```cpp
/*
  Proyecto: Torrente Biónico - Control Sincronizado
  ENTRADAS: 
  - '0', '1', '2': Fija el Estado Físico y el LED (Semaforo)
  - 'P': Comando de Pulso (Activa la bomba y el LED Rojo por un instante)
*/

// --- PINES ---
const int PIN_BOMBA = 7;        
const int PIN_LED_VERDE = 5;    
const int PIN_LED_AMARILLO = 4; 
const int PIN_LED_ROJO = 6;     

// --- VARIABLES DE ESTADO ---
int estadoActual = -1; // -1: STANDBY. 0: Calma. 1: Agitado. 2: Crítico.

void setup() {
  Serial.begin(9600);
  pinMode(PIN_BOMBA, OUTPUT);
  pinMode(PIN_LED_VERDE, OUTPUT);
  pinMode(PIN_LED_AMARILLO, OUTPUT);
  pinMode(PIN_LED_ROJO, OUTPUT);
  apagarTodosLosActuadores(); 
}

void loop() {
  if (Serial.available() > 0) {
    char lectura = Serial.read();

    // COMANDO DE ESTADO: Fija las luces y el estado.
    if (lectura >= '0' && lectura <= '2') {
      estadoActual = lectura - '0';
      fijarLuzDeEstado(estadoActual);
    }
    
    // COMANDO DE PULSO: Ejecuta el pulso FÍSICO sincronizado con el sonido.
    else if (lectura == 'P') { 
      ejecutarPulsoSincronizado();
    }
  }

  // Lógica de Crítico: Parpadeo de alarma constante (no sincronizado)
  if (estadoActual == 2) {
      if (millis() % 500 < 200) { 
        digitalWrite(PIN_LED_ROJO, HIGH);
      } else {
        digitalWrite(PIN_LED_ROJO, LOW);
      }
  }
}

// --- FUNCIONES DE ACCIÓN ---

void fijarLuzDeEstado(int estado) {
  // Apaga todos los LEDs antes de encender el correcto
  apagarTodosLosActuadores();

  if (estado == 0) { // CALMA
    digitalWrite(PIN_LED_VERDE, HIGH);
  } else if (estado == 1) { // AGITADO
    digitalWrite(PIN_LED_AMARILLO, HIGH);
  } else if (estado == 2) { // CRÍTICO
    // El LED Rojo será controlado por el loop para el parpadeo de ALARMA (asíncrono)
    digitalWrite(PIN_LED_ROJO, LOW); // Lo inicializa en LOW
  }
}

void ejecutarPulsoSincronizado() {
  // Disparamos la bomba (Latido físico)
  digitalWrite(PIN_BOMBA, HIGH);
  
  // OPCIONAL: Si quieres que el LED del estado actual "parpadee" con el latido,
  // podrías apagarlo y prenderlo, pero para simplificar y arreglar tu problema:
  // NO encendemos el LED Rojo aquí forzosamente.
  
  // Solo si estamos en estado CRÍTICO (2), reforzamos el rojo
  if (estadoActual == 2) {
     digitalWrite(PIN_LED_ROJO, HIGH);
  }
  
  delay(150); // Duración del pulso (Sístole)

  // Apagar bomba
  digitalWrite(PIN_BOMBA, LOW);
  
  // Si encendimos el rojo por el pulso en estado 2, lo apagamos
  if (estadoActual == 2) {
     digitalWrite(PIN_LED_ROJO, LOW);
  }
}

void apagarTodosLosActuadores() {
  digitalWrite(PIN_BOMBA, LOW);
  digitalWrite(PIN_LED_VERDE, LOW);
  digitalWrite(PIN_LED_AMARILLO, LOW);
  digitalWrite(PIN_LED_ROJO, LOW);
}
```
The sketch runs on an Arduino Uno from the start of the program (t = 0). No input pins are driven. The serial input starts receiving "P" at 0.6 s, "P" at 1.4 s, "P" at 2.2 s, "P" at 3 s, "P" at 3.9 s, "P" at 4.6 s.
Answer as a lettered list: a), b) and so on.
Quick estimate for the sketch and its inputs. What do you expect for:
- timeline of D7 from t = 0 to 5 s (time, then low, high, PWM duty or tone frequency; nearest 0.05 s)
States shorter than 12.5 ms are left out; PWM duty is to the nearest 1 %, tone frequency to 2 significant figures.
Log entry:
a) 0 s low; 0.6 s high; 0.75 s low; 1.4 s high; 1.55 s low; 2.2 s high; 2.35 s low; 3 s high; 3.15 s low; 3.9 s high; 4.05 s low; 4.6 s high; 4.75 s low
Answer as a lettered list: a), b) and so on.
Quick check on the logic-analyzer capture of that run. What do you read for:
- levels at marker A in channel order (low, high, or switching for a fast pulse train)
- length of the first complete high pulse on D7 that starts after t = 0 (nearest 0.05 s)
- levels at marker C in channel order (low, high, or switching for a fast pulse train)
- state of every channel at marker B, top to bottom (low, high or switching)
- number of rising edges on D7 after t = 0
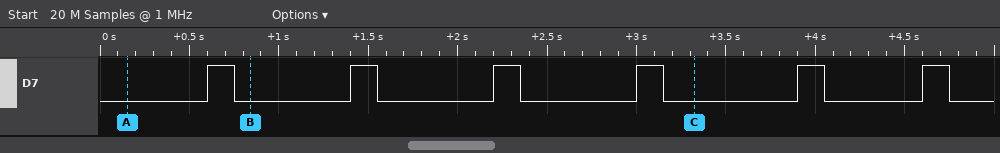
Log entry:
a) D7 low
b) 0.15 s
c) D7 low
d) D7 low
e) 6
